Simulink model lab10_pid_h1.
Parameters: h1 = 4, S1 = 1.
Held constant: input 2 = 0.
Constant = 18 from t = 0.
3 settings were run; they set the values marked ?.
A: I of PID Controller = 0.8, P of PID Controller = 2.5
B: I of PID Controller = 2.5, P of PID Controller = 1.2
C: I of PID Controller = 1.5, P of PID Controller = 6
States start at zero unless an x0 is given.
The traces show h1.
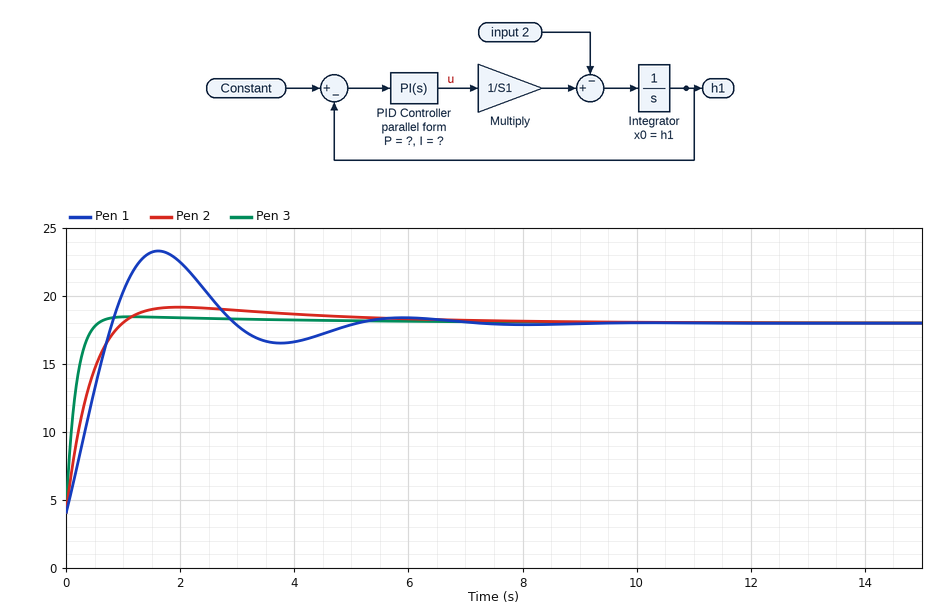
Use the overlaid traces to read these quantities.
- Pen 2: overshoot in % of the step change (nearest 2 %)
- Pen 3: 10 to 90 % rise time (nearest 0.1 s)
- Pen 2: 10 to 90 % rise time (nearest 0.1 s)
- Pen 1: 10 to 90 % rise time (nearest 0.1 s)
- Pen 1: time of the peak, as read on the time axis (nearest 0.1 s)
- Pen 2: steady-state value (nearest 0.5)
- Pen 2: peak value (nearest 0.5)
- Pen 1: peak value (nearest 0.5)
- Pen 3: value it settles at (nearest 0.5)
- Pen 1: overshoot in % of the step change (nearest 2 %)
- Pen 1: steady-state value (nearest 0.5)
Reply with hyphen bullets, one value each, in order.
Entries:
- 8 %
- 0.3 s
- 0.7 s
- 0.6 s
- 1.6 s
- 18.0
- 19.0
- 23.5
- 18.0
- 38 %
- 18.0
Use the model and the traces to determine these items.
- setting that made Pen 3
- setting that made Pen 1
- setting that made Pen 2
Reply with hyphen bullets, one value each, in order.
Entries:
- C
- B
- A
